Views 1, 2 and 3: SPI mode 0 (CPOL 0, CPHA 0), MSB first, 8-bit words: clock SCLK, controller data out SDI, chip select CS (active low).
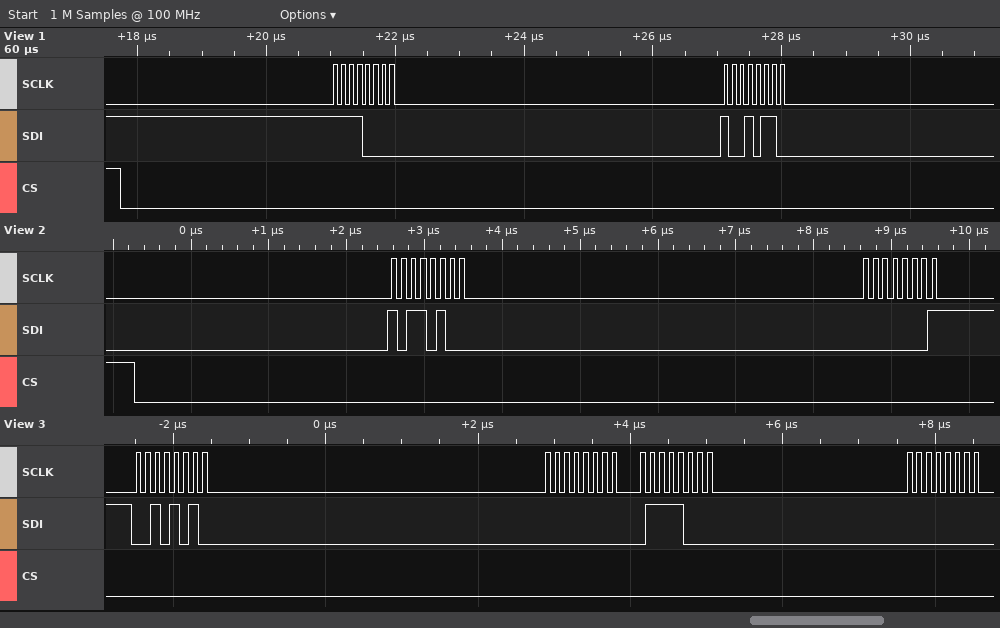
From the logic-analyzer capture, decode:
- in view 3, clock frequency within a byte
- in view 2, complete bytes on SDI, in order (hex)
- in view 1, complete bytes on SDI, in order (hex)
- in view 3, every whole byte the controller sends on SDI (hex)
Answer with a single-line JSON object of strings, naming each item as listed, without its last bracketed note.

{"in view 3, clock frequency within a byte": "8 MHz", "in view 2, complete bytes on SDI, in order": "0xB4 0x01", "in view 1, complete bytes on SDI, in order": "F0 96", "in view 3, every whole byte the controller sends on SDI": "2A 00 78 00"}
